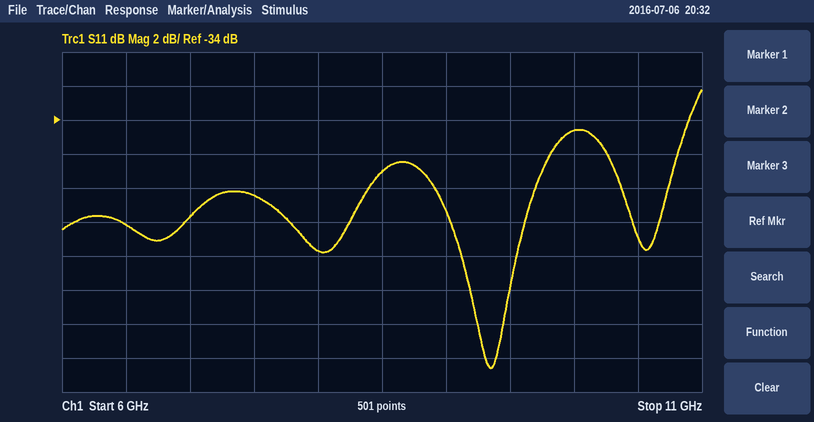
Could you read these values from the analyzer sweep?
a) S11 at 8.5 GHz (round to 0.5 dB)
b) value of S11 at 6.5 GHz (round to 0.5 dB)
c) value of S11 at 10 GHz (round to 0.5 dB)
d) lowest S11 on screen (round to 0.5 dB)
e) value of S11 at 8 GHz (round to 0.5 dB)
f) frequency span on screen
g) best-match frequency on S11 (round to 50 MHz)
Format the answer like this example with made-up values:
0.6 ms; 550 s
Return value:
-37.0 dB; -40.0 dB; -34.5 dB; -48.5 dB; -41.5 dB; 5 GHz; 9.35 GHz
